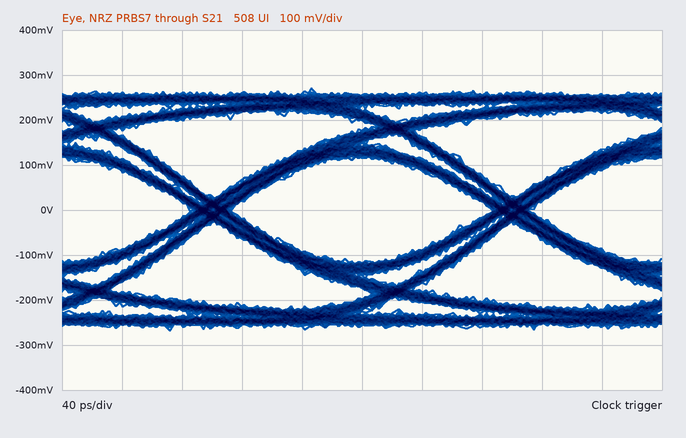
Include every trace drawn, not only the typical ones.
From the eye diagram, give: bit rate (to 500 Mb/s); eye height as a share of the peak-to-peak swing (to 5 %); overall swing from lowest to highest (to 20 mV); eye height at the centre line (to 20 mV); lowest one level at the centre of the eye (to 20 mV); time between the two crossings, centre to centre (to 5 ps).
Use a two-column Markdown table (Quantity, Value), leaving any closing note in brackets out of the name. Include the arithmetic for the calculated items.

| Quantity | Value |
|---|---|
| bit rate | 5.0 Gb/s |
| eye height as a share of the peak-to-peak swing | 240 mV / 540 mV ≈ 44.4 %, so 45 % to the nearest 5 % |
| overall swing from lowest to highest | 540 mV |
| eye height at the centre line | 240 mV |
| lowest one level at the centre of the eye | 120 mV |
| time between the two crossings, centre to centre | 200 ps |
